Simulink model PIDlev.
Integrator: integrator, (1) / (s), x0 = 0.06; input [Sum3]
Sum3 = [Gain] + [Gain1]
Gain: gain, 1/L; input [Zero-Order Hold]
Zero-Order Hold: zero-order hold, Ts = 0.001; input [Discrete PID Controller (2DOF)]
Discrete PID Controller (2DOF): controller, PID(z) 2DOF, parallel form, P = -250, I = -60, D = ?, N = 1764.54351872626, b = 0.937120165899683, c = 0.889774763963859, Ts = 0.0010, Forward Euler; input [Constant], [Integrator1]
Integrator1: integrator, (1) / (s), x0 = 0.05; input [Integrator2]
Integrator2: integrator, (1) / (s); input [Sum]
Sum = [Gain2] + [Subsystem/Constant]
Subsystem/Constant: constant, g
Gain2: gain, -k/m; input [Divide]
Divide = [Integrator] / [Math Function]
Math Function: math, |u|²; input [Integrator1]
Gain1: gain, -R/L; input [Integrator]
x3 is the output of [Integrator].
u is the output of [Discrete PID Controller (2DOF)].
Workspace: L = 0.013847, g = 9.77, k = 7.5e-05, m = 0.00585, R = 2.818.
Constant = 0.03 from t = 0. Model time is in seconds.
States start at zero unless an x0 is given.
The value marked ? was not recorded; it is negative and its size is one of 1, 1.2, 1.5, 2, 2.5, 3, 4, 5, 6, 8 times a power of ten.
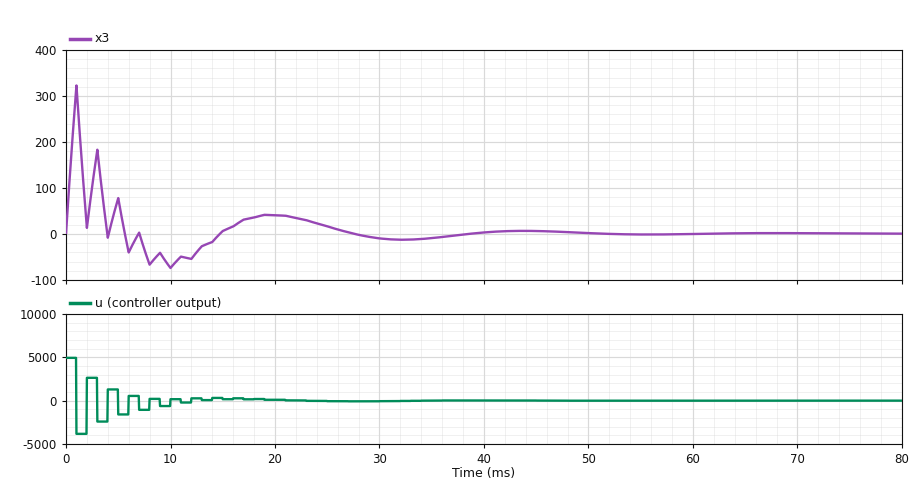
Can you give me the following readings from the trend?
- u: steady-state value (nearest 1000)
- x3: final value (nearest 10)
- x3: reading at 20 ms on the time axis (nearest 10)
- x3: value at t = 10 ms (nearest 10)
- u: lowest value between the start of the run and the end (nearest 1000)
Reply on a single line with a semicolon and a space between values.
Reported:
0; 0; 40; -70; -4000
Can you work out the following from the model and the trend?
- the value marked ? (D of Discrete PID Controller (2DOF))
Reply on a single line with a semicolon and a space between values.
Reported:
-120
